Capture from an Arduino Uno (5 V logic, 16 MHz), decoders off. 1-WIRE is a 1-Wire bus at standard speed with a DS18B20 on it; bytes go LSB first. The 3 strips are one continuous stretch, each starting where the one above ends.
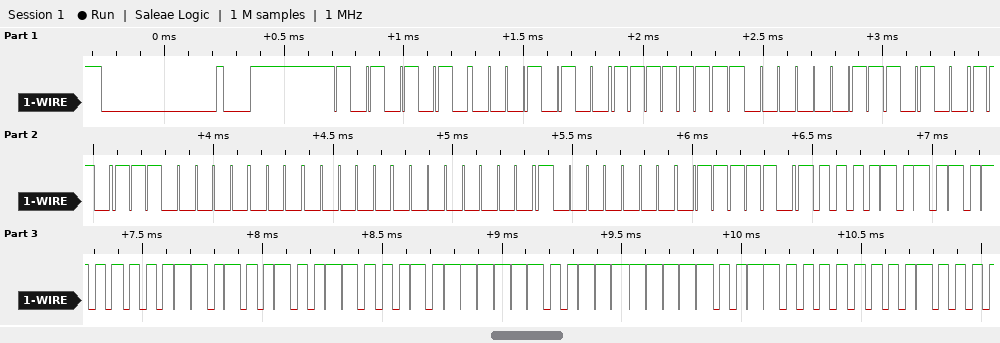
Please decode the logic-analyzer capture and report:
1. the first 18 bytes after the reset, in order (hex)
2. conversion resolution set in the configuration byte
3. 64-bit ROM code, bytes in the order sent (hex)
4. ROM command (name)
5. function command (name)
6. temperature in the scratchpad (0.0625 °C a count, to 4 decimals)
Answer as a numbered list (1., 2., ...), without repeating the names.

1. 55 28 FF C0 65 07 00 00 01 BE 50 05 4B 46 3F FF 0C 10
2. 10 bits
3. 28 FF C0 65 07 00 00 01
4. Match ROM
5. Read Scratchpad
6. 85.0000 °C
